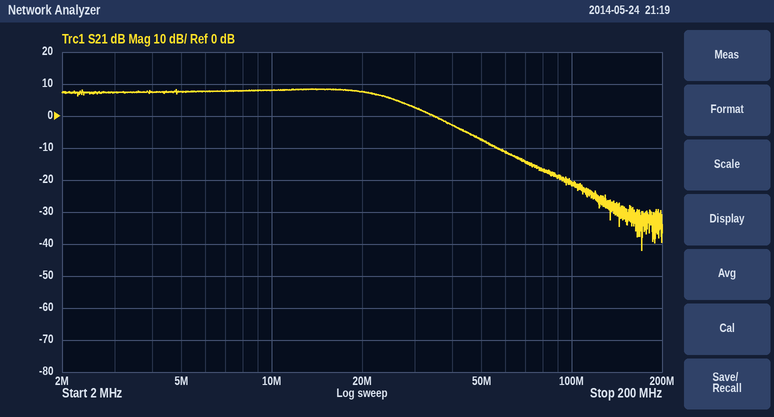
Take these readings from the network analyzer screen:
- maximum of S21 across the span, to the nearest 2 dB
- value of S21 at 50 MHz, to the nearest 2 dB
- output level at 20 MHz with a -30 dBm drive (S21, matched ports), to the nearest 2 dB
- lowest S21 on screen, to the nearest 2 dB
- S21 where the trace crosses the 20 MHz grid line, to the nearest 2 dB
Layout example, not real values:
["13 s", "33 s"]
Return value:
["8 dB", "-8 dB", "-22 dBm", "-42 dB", "8 dB"]
